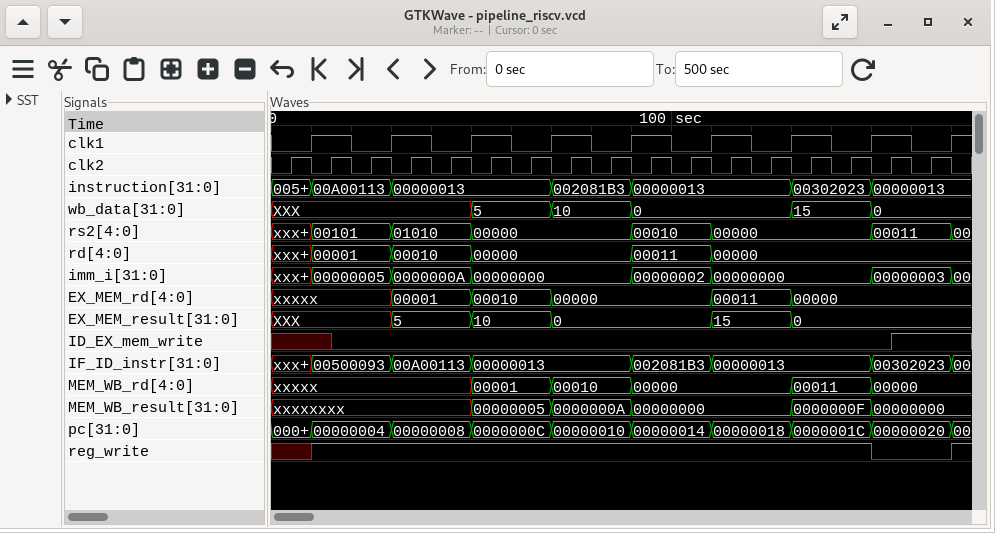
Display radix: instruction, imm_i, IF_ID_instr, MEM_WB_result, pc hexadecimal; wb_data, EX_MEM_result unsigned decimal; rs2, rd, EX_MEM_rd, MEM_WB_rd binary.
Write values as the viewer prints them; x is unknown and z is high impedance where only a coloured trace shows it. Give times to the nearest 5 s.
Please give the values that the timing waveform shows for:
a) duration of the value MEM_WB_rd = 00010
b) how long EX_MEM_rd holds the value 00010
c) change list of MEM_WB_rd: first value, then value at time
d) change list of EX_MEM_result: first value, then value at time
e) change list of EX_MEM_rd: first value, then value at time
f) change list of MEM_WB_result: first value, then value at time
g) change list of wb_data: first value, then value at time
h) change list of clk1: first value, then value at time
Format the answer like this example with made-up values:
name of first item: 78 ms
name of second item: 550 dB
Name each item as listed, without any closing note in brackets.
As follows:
duration of the value MEM_WB_rd = 00010: 20 s
how long EX_MEM_rd holds the value 00010: 20 s
change list of MEM_WB_rd: first value, then value at time: xxxxx, 00001 at 50 s, 00010 at 70 s, 00000 at 90 s, 00011 at 130 s, 00000 at 150 s
change list of EX_MEM_result: first value, then value at time: XXX, 5 at 30 s, 10 at 50 s, 0 at 70 s, 15 at 110 s, 0 at 130 s
change list of EX_MEM_rd: first value, then value at time: xxxxx, 00001 at 30 s, 00010 at 50 s, 00000 at 70 s, 00011 at 110 s, 00000 at 130 s
change list of MEM_WB_result: first value, then value at time: xxxxxxxx, 00000005 at 50 s, 0000000A at 70 s, 00000000 at 90 s, 0000000F at 130 s, 00000000 at 150 s
change list of wb_data: first value, then value at time: XXX, 5 at 50 s, 10 at 70 s, 0 at 90 s, 15 at 130 s, 0 at 150 s
change list of clk1: first value, then value at time: 0, 1 at 10 s, 0 at 20 s, 1 at 30 s, 0 at 40 s, 1 at 50 s, 0 at 60 s, 1 at 70 s, 0 at 80 s, 1 at 90 s, 0 at 100 s, 1 at 110 s, 0 at 120 s, 1 at 130 s, 0 at 140 s, 1 at 150 s, 0 at 160 s, 1 at 170 s
